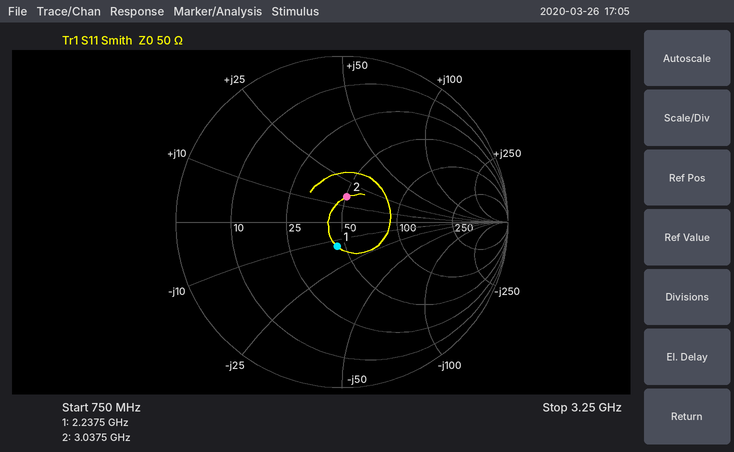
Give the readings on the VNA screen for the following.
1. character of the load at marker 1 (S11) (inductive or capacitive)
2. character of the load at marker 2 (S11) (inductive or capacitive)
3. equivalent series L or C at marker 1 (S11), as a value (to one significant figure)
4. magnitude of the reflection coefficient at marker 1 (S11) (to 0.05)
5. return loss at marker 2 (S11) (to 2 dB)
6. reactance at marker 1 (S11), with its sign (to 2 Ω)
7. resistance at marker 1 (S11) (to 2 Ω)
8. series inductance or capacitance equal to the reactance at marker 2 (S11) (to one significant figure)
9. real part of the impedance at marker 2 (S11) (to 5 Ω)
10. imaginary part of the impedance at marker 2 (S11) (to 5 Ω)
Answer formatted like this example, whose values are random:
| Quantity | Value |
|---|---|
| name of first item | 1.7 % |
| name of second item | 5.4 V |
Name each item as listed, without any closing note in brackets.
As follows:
| Quantity | Value |
|---|---|
| character of the load at marker 1 (S11) | capacitive |
| character of the load at marker 2 (S11) | inductive |
| equivalent series L or C at marker 1 (S11), as a value | 5 pF |
| magnitude of the reflection coefficient at marker 1 (S11) | 0.15 |
| return loss at marker 2 (S11) | 16 dB |
| reactance at marker 1 (S11), with its sign | -14 Ω |
| resistance at marker 1 (S11) | 46 Ω |
| series inductance or capacitance equal to the reactance at marker 2 (S11) | 800 pH |
| real part of the impedance at marker 2 (S11) | 50 Ω |
| imaginary part of the impedance at marker 2 (S11) | +15 Ω |
